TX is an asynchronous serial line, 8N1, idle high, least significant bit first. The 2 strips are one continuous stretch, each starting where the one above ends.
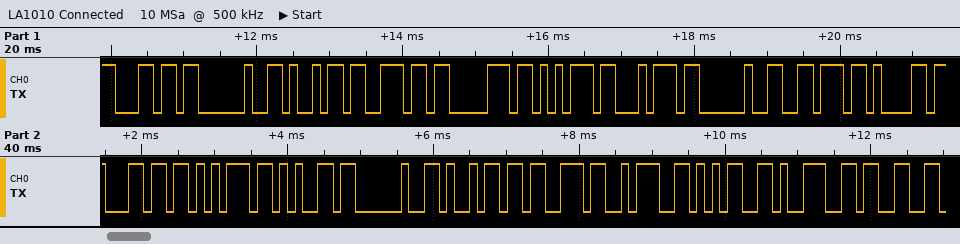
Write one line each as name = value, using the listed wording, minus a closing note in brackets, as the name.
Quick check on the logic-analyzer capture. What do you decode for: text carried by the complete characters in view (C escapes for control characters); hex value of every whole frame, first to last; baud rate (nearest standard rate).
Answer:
text carried by the complete characters in view = "l input value is:593"
hex value of every whole frame, first to last = 0x6C 0x20 0x69 0x6E 0x70 0x75 0x74 0x20 0x76 0x61 0x6C 0x75 0x65 0x20 0x69 0x73 0x3A 0x35 0x39 0x33
baud rate = 9600 baud
